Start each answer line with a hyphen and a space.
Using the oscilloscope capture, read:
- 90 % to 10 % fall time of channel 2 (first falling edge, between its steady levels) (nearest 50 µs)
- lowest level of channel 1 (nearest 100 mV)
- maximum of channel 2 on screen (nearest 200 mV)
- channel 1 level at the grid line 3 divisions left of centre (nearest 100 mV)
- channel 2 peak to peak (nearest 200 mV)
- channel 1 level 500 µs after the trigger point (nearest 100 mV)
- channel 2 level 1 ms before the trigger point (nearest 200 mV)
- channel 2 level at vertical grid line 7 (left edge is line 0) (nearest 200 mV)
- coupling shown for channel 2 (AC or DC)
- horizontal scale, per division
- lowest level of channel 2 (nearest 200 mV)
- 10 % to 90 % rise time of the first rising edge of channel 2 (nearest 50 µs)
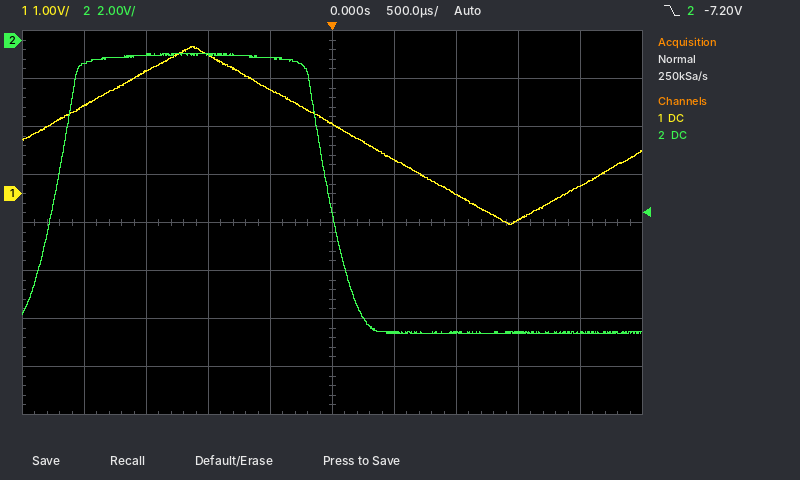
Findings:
- 400 µs
- -600 mV
- -600 mV
- 2.5 V
- 11.6 V
- 700 mV
- -600 mV
- -12.2 V
- DC
- 500 µs
- -12.2 V
- 400 µs
